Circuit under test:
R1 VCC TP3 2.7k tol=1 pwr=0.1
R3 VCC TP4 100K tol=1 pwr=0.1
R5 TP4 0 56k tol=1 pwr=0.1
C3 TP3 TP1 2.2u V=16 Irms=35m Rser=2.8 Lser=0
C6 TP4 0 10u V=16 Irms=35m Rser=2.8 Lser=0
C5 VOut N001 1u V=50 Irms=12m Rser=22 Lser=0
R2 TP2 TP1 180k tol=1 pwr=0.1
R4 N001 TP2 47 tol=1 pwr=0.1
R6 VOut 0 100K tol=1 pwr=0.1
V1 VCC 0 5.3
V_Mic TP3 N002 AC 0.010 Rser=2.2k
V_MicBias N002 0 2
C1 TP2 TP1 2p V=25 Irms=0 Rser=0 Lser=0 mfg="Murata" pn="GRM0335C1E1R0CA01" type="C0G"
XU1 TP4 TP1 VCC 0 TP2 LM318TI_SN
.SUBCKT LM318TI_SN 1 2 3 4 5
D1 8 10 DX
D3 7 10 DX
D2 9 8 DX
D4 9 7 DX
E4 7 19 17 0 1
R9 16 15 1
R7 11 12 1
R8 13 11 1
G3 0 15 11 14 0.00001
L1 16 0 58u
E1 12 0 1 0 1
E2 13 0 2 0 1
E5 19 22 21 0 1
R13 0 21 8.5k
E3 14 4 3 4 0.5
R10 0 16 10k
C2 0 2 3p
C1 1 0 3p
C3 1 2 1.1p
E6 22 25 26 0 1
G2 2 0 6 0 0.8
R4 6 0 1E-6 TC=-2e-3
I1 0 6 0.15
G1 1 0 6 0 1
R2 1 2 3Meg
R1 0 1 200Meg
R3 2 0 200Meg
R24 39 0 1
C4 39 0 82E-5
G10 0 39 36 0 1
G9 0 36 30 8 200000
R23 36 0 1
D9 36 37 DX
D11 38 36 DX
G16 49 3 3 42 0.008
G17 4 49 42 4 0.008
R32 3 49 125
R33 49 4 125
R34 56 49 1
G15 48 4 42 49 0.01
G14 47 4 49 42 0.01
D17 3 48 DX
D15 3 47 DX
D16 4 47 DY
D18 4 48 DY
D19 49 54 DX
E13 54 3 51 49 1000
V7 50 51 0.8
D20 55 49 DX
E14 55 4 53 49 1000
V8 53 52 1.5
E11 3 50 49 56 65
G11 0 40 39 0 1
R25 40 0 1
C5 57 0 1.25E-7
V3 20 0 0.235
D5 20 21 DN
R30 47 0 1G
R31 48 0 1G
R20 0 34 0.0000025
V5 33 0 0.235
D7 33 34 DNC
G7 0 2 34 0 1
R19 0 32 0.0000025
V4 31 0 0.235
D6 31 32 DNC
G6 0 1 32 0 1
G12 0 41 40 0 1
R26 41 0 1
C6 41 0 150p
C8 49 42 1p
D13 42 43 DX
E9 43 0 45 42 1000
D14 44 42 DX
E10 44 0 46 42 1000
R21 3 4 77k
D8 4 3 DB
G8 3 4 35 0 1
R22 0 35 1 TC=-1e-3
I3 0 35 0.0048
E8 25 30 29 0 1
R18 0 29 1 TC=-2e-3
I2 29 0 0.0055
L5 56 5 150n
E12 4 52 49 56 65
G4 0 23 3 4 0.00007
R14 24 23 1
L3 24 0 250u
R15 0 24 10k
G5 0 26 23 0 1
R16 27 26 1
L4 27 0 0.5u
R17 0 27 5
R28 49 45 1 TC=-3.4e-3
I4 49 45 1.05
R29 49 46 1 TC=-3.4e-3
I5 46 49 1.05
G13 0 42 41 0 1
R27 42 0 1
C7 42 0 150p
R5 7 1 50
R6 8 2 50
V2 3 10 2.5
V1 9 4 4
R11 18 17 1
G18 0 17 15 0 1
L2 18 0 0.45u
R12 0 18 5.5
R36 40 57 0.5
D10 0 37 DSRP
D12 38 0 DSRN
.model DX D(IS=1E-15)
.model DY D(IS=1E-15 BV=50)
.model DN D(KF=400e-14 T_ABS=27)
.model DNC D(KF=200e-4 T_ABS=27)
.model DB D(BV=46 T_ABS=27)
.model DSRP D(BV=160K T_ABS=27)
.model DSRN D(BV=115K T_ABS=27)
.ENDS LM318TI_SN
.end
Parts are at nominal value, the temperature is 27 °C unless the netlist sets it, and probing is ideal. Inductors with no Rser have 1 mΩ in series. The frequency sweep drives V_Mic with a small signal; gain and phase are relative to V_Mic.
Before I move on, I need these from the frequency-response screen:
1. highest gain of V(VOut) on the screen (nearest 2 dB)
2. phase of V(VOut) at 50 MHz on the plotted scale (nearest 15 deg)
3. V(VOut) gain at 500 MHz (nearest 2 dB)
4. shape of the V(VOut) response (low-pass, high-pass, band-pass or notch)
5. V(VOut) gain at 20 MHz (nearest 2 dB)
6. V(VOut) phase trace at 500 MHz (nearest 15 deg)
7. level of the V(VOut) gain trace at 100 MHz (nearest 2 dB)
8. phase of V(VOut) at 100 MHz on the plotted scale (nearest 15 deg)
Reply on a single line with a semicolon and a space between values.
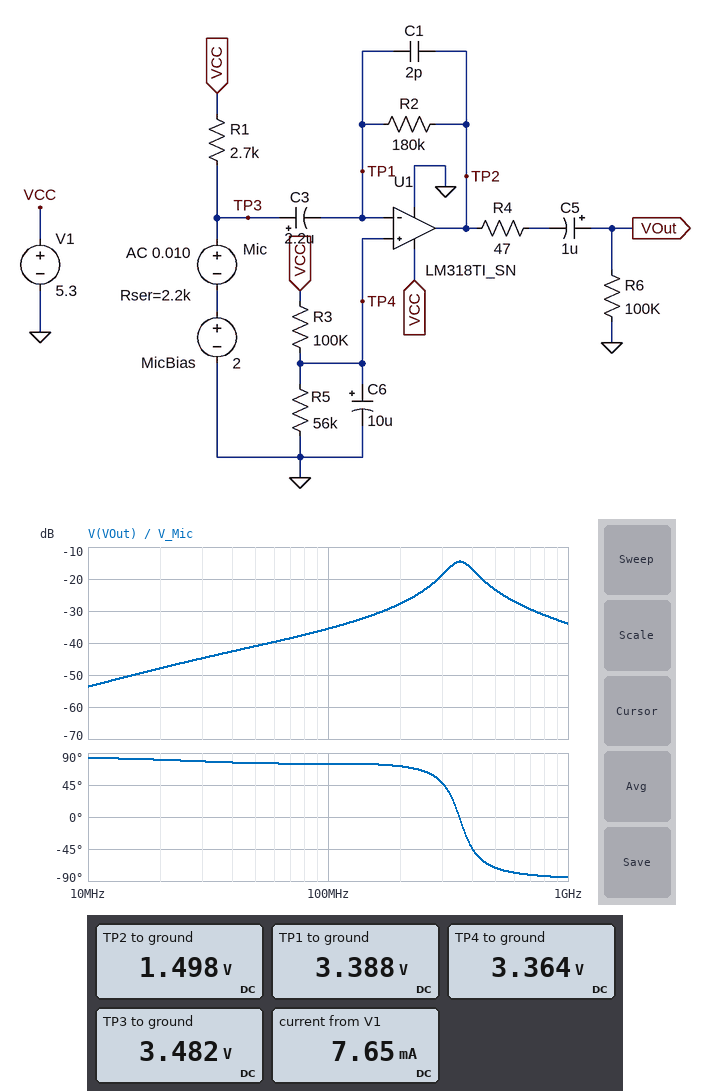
-14 dB; 75 deg; -24 dB; band-pass; -48 dB; -75 deg; -36 dB; 75 deg
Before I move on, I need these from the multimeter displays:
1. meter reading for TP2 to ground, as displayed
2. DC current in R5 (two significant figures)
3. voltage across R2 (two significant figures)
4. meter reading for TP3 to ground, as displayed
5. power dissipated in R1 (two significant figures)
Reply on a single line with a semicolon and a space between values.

1.498 V; 60 µA; 1.9 V; 3.482 V; 1.2 mW
